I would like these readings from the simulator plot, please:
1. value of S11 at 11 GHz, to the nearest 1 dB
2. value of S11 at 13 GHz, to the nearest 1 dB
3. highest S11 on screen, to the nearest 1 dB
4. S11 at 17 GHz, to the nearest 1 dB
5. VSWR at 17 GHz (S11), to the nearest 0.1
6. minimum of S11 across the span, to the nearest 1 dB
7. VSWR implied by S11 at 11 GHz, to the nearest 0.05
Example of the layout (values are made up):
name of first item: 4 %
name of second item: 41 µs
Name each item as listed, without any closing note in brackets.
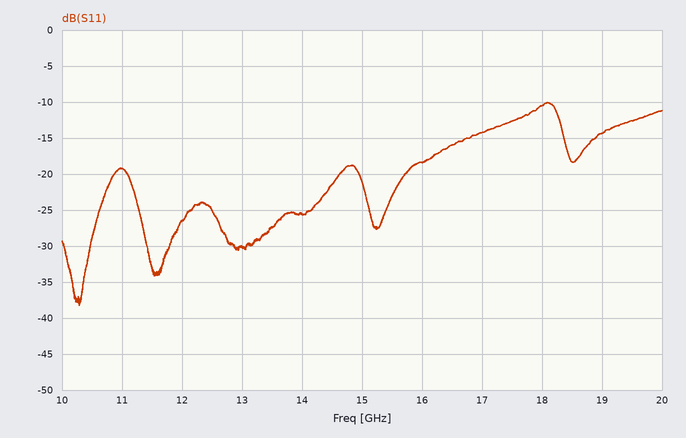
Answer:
value of S11 at 11 GHz, to the nearest 1 dB: -19 dB
value of S11 at 13 GHz, to the nearest 1 dB: -30 dB
highest S11 on screen, to the nearest 1 dB: -10 dB
S11 at 17 GHz, to the nearest 1 dB: -14 dB
VSWR at 17 GHz (S11), to the nearest 0.1: 1.5
minimum of S11 across the span, to the nearest 1 dB: -38 dB
VSWR implied by S11 at 11 GHz, to the nearest 0.05: 1.25
